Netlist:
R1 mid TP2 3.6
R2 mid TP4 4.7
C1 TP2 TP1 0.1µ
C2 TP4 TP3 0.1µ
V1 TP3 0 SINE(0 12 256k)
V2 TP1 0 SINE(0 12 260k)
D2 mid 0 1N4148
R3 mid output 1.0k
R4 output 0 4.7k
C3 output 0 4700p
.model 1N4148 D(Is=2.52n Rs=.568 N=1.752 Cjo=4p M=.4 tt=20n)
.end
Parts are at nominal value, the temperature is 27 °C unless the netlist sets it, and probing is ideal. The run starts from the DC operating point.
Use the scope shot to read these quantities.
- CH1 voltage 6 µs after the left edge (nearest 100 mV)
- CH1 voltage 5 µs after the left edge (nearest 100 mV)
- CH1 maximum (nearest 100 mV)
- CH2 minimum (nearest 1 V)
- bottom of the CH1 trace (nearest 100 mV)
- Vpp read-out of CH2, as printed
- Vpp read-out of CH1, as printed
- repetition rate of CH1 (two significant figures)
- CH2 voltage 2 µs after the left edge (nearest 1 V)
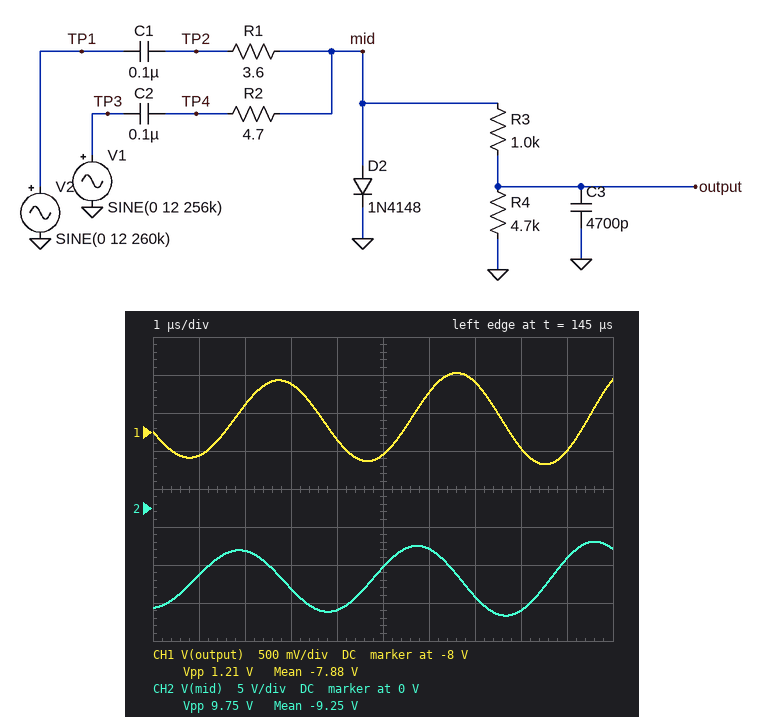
-7.5 V
-8.3 V
-7.2 V
-14 V
-8.4 V
9.75 V
1.21 V
260 kHz
-6 V
